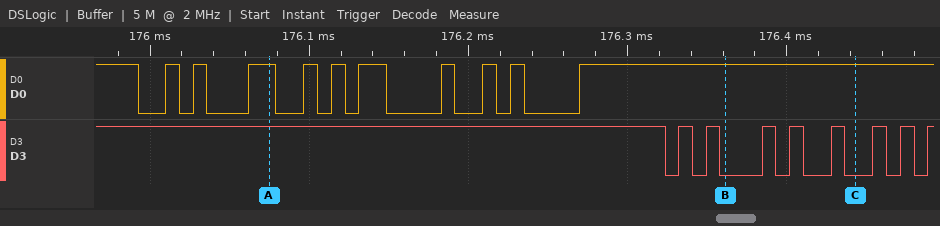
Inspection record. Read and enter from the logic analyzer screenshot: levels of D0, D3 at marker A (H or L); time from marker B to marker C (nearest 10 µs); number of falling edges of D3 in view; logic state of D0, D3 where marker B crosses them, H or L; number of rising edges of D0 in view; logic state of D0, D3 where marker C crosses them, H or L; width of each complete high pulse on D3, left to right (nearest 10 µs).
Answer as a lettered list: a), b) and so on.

a) D0=H, D3=H
b) 80 µs
c) 8
d) D0=H, D3=L
e) 10
f) D0=H, D3=L
g) 10 µs, 10 µs, 10 µs, 10 µs, 10 µs, 10 µs, 10 µs
